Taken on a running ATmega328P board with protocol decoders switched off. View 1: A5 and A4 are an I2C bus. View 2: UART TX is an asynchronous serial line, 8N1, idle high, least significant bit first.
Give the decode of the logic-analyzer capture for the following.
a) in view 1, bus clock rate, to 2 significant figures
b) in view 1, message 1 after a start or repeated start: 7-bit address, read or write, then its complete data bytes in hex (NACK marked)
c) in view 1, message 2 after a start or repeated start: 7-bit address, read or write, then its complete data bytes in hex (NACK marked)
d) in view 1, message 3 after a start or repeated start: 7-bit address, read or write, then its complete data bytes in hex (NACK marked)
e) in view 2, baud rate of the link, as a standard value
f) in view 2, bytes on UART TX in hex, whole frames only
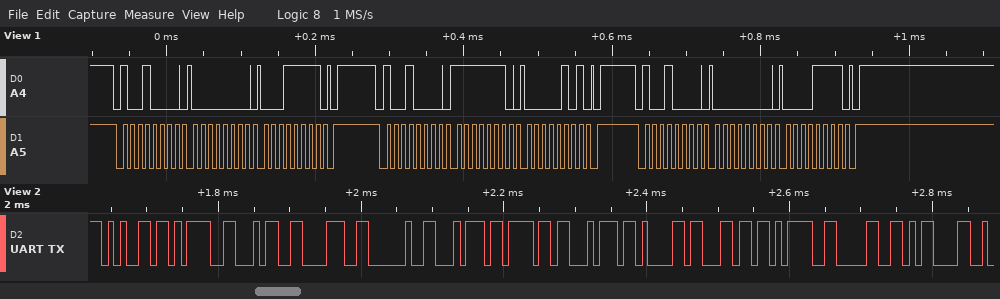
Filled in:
100 kHz
0x48 write: 00 1F
0x48 write: FE 05
0x48 write: 00 0F
115200 baud
65 3D 34 38 20 74 6F 74 61 6C 3D 30 0D
